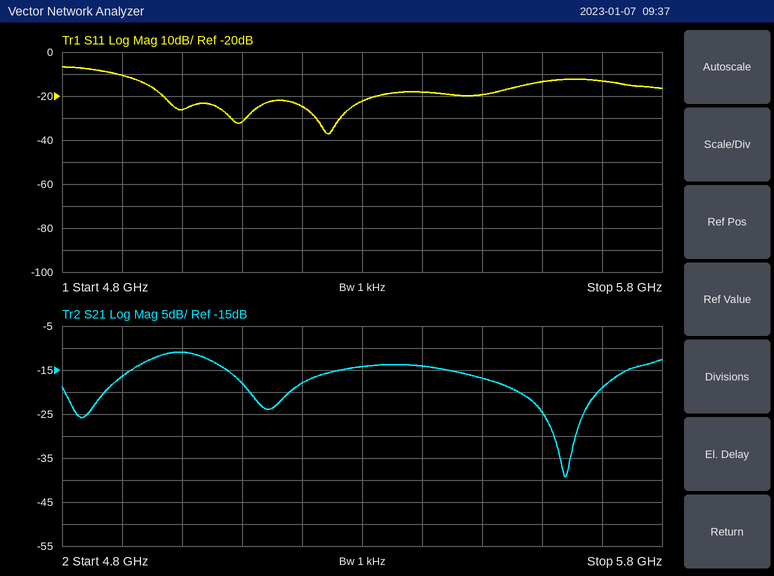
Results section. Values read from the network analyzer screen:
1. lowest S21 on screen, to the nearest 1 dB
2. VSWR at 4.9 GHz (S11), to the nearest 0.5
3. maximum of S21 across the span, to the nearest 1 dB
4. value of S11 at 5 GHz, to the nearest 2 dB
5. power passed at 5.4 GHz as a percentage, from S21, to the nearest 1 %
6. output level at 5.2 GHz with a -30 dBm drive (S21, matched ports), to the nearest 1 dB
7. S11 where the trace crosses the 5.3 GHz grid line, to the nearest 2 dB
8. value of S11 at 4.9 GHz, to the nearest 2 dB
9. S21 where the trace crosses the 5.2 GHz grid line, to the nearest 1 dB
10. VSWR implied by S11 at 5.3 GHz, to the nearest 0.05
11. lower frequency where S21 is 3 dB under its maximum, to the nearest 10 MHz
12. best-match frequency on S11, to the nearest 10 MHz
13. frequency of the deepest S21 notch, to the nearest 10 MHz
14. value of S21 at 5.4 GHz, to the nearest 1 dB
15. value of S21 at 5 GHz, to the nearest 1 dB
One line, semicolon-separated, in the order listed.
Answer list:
-39 dB; 2.0; -11 dB; -26 dB; 4 %; -48 dBm; -22 dB; -10 dB; -18 dB; 1.15; 4.93 GHz; 5.24 GHz; 5.64 GHz; -14 dB; -11 dB
